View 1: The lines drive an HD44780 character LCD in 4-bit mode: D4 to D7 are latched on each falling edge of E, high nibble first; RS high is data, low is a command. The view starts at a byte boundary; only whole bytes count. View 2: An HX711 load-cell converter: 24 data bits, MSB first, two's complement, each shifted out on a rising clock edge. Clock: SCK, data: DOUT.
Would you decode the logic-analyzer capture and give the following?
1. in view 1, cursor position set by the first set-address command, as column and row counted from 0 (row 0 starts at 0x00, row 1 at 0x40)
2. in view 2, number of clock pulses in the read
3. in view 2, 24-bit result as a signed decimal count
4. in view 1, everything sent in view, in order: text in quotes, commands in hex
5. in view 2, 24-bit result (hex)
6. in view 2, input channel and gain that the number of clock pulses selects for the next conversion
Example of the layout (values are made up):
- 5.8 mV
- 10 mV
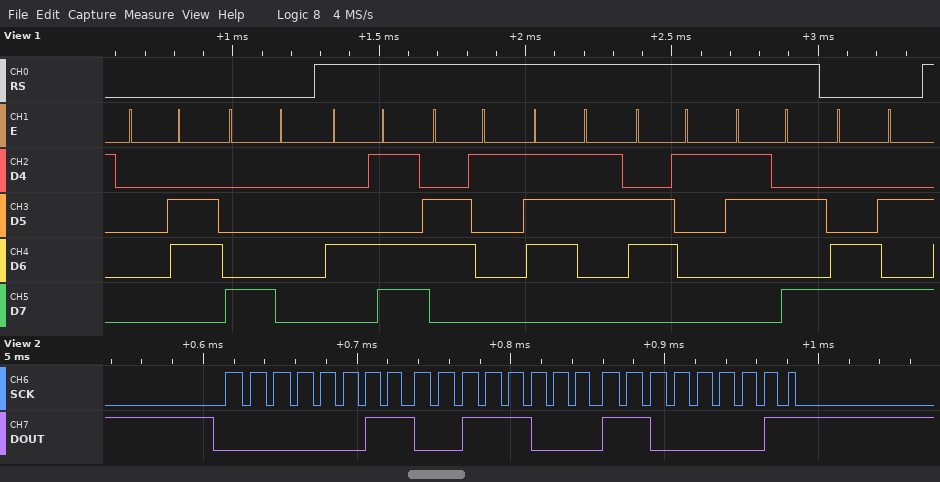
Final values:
- column 0, row 0
- 25
- 211137
- 0x06 0x80 "Masa:" 0xCA
- 0x0338C1
- channel A, gain 128
